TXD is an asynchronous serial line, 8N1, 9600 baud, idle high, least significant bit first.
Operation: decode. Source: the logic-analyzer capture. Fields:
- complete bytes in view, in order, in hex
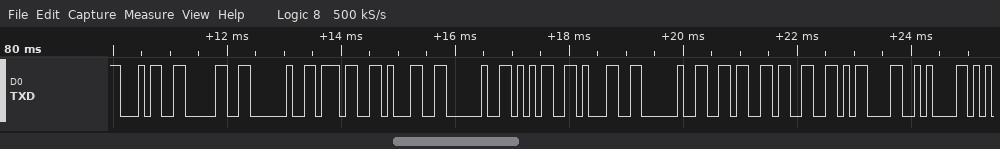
0x34 0x30 0x20 0x37 0x31 0x20 0x35 0x31 0x20 0x36 0x33 0x0D 0x0A
